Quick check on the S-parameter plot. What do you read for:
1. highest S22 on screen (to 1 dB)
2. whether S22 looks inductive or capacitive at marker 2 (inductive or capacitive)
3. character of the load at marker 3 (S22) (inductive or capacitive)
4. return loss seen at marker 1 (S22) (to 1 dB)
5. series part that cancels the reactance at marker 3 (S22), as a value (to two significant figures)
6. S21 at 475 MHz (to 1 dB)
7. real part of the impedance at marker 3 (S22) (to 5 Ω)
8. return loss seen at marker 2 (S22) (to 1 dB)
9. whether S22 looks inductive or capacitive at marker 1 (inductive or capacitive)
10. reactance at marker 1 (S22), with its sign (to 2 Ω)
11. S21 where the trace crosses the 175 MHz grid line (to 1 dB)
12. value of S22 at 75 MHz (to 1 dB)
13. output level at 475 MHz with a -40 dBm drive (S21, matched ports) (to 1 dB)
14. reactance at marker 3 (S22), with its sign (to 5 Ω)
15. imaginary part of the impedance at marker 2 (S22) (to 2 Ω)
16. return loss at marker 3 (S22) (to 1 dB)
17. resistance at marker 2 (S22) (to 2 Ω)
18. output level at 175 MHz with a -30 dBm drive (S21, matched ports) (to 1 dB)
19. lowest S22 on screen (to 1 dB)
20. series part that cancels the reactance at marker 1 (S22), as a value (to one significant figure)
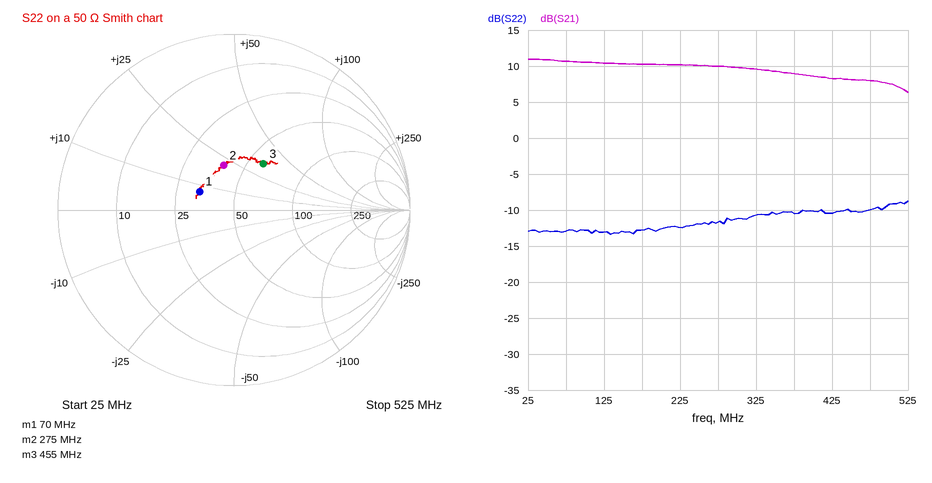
-9 dB
inductive
inductive
13 dB
10 pF
8 dB
60 Ω
12 dB
inductive
+8 Ω
10 dB
-13 dB
-32 dBm
+35 Ω
+22 Ω
10 dB
40 Ω
-20 dBm
-13 dB
300 pF
